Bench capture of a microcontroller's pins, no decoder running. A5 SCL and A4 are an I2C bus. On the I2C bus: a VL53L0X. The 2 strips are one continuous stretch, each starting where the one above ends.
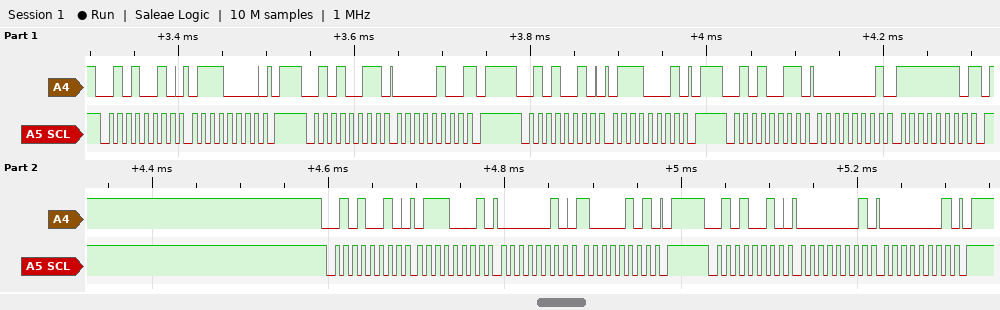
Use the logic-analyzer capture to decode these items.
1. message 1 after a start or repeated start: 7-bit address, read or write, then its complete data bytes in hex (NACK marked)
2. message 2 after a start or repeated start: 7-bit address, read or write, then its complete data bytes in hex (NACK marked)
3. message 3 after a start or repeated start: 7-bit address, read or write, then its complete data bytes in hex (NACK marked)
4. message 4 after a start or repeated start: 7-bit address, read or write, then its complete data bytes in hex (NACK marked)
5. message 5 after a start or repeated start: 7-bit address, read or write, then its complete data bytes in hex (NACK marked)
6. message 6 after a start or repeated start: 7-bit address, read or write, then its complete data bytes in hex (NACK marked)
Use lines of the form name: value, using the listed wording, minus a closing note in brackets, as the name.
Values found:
message 1 after a start or repeated start: 7-bit address, read or write, then its complete data bytes in hex: 0x29 write: 70
message 2 after a start or repeated start: 7-bit address, read or write, then its complete data bytes in hex: 0x29 read: 04 NACK
message 3 after a start or repeated start: 7-bit address, read or write, then its complete data bytes in hex: 0x29 write: 71
message 4 after a start or repeated start: 7-bit address, read or write, then its complete data bytes in hex: 0x29 read: 01 FE NACK
message 5 after a start or repeated start: 7-bit address, read or write, then its complete data bytes in hex: 0x29 write: 71 02 85
message 6 after a start or repeated start: 7-bit address, read or write, then its complete data bytes in hex: 0x29 write: 01 01
